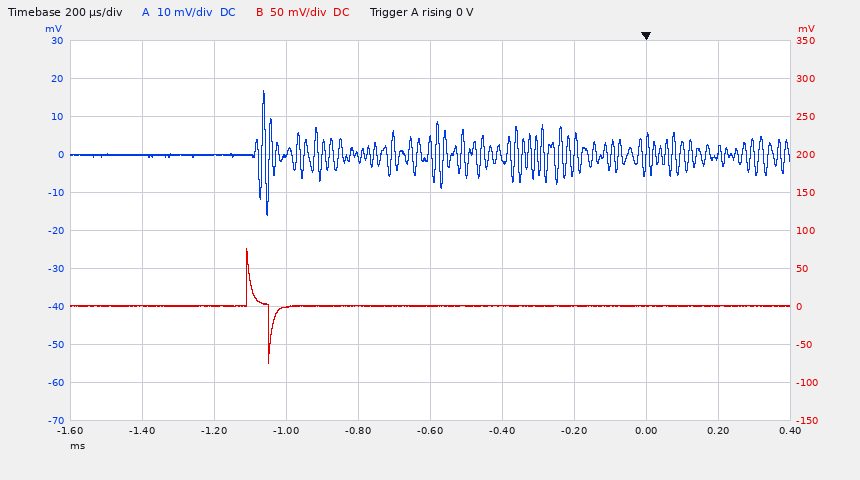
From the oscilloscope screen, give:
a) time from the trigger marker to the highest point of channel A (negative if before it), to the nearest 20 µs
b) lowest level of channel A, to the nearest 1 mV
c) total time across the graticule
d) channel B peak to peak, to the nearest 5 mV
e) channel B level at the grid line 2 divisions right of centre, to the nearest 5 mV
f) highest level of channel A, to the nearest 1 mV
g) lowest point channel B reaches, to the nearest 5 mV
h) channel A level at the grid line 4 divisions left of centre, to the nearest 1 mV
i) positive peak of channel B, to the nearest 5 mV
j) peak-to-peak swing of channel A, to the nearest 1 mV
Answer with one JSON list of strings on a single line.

["-1.06 ms", "-16 mV", "2 ms", "150 mV", "0 mV", "17 mV", "-75 mV", "0 mV", "75 mV", "33 mV"]
